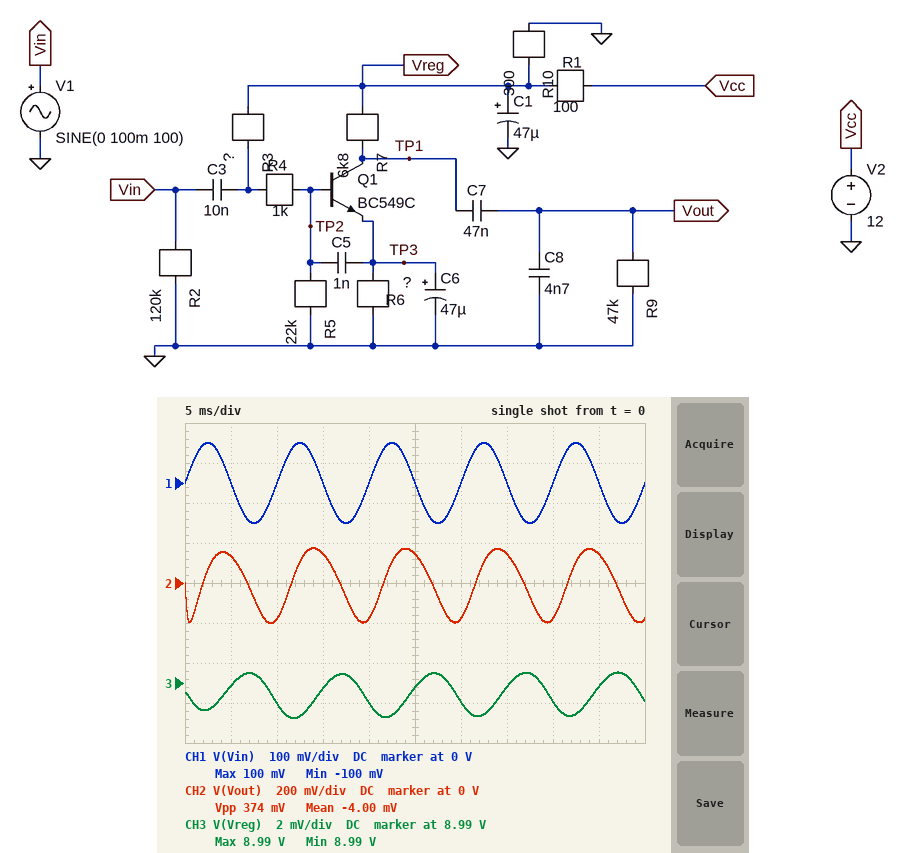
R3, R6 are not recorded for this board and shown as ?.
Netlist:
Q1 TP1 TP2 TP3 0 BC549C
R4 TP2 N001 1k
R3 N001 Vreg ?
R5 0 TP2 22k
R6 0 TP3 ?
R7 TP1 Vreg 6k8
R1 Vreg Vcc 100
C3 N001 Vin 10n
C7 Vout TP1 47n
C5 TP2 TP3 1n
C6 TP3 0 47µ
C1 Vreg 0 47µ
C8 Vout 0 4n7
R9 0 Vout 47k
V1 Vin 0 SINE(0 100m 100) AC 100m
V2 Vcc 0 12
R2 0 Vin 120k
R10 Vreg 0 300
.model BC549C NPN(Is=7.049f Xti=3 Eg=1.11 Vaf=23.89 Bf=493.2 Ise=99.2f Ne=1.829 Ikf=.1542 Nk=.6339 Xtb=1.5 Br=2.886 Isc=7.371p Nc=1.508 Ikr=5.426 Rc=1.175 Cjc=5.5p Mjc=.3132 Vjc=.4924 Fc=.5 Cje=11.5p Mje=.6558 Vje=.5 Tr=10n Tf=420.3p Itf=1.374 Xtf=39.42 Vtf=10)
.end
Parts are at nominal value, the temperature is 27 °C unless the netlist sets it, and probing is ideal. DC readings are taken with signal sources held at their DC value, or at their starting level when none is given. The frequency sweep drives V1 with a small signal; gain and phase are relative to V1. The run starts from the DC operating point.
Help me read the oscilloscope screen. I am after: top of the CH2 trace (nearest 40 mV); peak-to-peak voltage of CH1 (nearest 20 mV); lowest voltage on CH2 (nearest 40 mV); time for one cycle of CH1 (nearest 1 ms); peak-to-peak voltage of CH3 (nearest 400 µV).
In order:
160 mV
200 mV
-200 mV
10 ms
2.4 mV
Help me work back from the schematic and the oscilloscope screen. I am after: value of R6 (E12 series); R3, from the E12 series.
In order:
3.9 kΩ
180 kΩ
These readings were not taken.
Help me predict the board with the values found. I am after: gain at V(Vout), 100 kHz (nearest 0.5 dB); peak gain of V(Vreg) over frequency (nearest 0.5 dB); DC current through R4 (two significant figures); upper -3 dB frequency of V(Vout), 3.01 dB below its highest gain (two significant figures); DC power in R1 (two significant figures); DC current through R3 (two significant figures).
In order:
-0.5 dB
-39.0 dB
44 µA
7.7 kHz
91 mW
44 µA
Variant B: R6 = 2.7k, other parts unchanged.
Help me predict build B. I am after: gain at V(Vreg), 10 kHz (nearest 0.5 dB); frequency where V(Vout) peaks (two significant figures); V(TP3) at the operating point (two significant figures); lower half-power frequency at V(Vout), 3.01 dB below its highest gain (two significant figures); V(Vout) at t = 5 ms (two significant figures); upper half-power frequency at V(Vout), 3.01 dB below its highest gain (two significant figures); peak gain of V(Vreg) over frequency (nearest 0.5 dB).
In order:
-63.0 dB
2.3 kHz
360 mV
670 Hz
170 mV
7.8 kHz
-36.5 dB
